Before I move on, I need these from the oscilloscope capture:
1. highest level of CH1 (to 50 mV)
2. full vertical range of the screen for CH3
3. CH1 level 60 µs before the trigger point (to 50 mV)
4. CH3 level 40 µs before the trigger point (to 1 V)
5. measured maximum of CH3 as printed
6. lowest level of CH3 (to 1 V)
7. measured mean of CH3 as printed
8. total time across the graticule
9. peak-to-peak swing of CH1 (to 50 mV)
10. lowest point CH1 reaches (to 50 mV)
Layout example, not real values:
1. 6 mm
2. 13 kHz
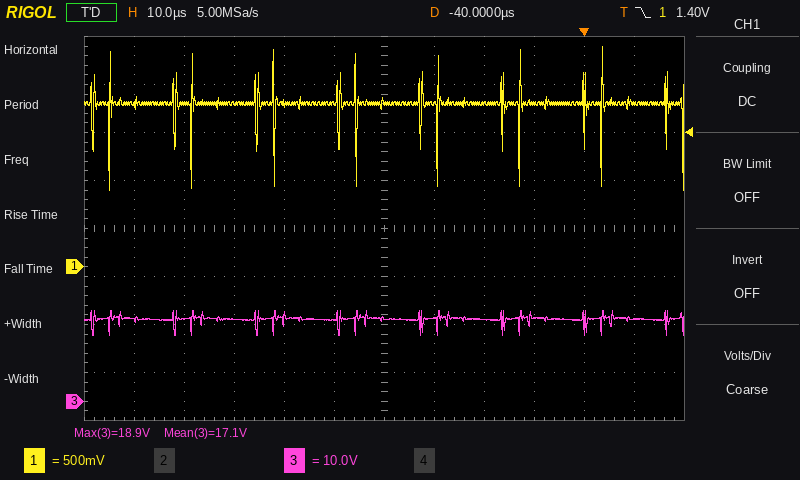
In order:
1. 2.30 V
2. 80 V
3. 1.70 V
4. 17 V
5. 18.9 V
6. 14 V
7. 17.1 V
8. 120 µs
9. 1.50 V
10. 800 mV
